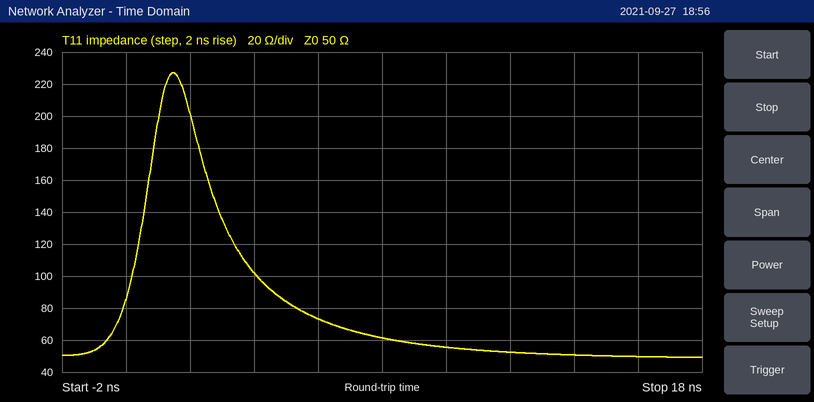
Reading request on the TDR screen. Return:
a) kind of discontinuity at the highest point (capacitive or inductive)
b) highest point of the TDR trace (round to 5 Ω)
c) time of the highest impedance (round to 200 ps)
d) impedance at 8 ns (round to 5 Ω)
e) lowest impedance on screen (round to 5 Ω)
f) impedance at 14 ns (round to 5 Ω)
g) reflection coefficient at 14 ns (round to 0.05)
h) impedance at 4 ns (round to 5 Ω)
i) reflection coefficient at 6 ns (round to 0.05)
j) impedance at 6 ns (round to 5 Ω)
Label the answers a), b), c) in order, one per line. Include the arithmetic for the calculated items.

a) inductive
b) 225 Ω
c) 1.4 ns
d) 60 Ω
e) 50 Ω
f) 50 Ω
g) (50 − 50)/(50 + 50) ≈ 0.00
h) 100 Ω
i) (75 − 50)/(75 + 50) ≈ +0.20
j) 75 Ω
